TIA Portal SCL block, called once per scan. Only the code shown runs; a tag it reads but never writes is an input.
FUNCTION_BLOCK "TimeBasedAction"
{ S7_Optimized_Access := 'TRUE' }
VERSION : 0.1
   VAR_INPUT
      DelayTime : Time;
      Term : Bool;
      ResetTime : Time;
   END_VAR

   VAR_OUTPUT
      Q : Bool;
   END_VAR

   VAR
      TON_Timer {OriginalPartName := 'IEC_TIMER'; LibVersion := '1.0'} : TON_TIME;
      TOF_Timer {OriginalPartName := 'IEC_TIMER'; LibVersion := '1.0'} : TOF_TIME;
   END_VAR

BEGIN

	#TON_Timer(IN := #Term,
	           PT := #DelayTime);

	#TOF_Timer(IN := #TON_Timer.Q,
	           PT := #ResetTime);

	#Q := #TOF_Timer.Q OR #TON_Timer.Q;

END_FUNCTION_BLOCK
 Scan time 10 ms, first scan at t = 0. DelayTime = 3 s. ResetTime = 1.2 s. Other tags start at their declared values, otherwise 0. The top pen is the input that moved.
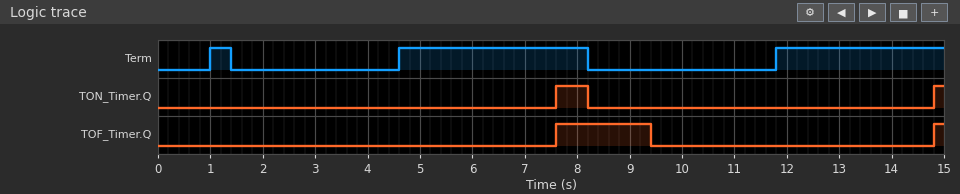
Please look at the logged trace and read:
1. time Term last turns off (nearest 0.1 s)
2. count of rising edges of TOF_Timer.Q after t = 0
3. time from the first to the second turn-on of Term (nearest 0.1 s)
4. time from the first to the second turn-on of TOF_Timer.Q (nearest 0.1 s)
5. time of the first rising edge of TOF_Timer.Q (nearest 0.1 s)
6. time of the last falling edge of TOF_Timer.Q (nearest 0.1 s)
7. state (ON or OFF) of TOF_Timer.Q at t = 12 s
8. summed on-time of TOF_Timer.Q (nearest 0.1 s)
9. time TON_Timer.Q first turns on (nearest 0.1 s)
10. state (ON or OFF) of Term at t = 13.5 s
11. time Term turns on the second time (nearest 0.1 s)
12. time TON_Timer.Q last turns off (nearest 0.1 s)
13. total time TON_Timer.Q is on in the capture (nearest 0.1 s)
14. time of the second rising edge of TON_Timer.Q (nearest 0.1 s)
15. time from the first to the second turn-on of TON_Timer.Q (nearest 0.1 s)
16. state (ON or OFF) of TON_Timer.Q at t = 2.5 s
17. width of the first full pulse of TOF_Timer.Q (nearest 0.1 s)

8.2 s
2
3.6 s
7.2 s
7.6 s
9.4 s
OFF
2.0 s
7.6 s
ON
4.6 s
8.2 s
0.8 s
14.8 s
7.2 s
OFF
1.8 s
